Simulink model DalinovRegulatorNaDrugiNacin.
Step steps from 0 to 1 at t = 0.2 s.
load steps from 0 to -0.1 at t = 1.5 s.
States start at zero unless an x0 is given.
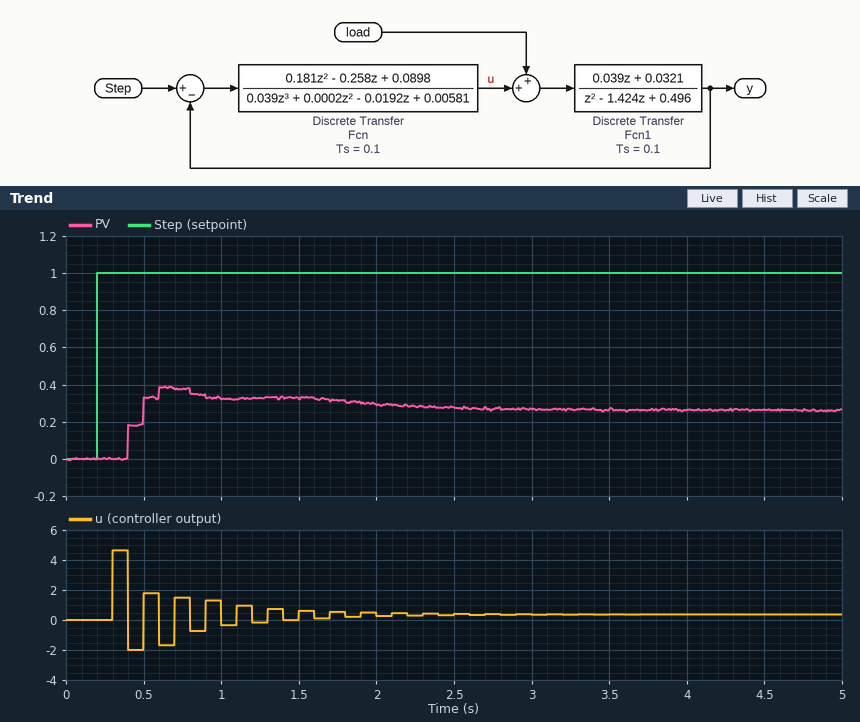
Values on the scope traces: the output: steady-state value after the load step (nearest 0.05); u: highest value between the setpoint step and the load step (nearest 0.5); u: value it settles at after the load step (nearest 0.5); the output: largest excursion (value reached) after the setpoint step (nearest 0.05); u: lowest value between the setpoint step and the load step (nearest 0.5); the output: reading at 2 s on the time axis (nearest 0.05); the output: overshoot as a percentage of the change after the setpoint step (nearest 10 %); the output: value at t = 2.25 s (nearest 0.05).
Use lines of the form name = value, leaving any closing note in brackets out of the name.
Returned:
the output: steady-state value after the load step = 0.25
u: highest value between the setpoint step and the load step = 4.5
u: value it settles at after the load step = 0.5
the output: largest excursion (value reached) after the setpoint step = 0.40
u: lowest value between the setpoint step and the load step = -2.0
the output: reading at 2 s on the time axis = 0.30
the output: overshoot as a percentage of the change after the setpoint step = 20 %
the output: value at t = 2.25 s = 0.30
